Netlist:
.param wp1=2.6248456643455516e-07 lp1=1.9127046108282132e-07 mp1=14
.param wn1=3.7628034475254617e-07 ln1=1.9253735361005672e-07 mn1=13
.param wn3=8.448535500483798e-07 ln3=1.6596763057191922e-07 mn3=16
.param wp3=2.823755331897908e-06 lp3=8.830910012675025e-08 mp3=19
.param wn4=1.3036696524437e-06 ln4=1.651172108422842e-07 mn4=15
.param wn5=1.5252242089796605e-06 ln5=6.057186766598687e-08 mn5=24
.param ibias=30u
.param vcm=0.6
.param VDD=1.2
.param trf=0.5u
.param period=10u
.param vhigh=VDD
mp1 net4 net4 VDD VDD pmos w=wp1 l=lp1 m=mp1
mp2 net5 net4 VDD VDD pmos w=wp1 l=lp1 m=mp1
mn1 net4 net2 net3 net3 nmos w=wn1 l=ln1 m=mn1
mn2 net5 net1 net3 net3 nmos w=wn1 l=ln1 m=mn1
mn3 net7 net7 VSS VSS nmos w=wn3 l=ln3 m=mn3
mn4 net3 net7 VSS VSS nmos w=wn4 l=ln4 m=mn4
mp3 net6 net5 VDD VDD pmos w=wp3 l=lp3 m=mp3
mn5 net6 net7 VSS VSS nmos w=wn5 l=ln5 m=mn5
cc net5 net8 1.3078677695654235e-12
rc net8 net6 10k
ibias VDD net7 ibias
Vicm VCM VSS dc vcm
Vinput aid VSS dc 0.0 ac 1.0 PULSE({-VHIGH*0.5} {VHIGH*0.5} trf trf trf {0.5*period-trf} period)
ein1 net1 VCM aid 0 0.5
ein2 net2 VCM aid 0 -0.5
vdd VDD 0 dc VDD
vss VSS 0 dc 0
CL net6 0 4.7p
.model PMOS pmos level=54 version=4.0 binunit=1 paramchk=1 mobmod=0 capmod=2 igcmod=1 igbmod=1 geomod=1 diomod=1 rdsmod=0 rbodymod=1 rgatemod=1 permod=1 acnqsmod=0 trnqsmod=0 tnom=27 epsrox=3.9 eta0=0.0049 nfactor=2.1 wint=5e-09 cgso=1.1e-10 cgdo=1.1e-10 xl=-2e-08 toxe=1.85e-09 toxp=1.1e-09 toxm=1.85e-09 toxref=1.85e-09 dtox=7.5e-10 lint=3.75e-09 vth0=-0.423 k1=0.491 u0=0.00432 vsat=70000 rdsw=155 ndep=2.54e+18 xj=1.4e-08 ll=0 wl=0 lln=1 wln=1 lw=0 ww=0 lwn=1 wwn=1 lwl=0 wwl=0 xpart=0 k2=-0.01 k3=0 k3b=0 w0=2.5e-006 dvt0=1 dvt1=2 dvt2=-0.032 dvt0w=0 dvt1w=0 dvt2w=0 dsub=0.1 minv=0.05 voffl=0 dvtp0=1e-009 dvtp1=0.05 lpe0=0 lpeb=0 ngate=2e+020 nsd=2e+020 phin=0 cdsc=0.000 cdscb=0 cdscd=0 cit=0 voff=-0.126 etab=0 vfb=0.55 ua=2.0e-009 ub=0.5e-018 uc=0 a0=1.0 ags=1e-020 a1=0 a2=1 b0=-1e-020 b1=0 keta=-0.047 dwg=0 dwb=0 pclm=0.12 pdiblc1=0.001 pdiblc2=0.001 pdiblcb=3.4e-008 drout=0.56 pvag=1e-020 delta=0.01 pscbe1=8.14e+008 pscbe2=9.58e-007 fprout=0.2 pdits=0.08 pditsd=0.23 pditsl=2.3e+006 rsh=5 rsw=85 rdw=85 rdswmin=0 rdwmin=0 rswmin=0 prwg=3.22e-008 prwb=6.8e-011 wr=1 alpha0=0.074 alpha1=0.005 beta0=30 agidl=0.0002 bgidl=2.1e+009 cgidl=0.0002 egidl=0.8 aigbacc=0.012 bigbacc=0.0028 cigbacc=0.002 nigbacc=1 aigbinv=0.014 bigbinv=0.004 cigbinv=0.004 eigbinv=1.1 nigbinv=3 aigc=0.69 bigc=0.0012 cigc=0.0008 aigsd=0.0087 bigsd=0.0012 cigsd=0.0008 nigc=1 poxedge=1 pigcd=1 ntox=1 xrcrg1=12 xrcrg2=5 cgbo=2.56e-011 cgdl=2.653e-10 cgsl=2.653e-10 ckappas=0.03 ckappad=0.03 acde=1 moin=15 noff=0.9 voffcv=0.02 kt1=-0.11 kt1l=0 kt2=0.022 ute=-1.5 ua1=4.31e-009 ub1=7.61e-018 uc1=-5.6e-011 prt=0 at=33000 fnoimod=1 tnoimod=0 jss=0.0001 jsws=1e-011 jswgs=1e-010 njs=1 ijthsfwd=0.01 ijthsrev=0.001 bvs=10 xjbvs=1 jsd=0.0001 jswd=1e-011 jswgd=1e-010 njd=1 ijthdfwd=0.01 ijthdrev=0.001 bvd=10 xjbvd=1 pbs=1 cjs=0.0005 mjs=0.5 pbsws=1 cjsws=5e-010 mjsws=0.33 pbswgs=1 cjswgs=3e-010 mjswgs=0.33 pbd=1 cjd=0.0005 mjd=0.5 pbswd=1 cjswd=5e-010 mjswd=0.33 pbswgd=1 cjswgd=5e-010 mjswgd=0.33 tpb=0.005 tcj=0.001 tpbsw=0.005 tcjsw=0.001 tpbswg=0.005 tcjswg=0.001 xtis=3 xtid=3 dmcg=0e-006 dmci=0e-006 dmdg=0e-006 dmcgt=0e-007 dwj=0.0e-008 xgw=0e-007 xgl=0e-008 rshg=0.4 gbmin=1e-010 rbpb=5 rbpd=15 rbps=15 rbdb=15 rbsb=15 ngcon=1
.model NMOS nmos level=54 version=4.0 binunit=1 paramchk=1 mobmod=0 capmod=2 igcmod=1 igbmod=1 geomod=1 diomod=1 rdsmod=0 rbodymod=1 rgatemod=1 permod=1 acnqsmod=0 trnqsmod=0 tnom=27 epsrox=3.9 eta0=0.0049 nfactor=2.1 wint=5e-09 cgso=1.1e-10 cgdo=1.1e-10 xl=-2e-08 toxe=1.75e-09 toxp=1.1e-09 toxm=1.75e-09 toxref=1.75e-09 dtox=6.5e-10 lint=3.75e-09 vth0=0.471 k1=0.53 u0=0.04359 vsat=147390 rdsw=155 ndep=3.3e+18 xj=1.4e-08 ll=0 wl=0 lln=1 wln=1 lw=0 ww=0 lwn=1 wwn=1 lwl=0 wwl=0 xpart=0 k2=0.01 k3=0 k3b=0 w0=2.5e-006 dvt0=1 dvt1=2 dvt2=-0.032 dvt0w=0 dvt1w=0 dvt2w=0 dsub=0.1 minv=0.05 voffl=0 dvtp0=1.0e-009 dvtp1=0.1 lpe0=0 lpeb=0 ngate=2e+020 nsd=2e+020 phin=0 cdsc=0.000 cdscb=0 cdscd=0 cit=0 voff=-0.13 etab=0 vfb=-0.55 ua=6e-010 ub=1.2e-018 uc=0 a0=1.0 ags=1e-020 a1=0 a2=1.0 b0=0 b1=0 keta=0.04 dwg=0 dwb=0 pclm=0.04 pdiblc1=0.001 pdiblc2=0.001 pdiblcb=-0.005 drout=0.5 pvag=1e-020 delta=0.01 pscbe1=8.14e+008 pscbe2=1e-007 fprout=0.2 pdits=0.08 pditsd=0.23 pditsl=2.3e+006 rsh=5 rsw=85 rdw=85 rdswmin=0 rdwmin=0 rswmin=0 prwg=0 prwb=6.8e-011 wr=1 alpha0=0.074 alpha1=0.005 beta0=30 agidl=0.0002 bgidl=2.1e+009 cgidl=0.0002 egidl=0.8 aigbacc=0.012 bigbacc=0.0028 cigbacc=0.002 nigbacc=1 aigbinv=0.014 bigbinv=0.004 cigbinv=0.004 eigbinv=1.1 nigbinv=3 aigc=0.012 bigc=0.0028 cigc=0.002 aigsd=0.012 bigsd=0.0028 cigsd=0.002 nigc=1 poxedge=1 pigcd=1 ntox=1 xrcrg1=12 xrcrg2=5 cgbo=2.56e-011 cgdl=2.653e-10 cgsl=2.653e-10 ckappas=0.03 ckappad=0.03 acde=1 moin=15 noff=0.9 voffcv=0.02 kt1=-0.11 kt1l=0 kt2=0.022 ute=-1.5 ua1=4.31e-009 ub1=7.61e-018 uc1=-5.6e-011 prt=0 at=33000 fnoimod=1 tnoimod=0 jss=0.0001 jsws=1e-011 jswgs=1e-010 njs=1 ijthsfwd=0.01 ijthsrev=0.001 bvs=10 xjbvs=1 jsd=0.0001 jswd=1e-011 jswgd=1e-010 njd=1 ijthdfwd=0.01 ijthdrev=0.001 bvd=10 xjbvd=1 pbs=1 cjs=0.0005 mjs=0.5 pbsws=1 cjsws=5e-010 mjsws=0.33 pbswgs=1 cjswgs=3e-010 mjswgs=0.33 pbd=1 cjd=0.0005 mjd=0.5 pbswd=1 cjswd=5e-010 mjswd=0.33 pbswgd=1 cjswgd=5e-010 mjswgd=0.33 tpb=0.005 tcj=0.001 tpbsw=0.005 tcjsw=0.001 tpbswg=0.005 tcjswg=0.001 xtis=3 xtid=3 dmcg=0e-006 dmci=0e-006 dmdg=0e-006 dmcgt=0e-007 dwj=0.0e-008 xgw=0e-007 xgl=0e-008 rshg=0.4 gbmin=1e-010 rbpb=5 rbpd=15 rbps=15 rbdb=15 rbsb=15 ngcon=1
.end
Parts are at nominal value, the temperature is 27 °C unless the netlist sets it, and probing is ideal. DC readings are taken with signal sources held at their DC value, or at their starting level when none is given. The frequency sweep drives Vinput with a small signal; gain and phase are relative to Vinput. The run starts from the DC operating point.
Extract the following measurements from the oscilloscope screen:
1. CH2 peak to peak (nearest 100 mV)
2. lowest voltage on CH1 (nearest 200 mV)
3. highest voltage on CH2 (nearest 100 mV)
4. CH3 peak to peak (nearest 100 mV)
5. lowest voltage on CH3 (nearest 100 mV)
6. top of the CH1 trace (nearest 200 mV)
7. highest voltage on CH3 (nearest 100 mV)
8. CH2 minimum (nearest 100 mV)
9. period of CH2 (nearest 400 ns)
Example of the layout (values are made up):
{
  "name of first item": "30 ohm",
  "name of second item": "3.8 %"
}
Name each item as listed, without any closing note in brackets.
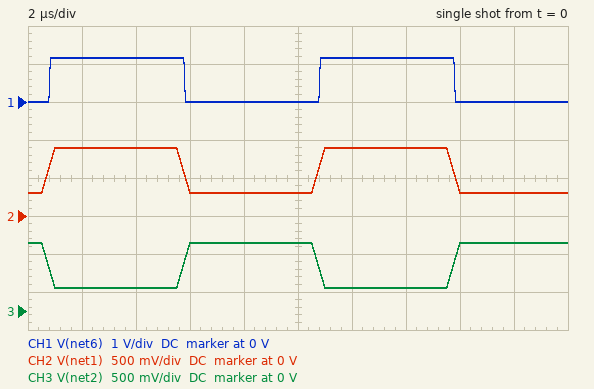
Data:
{
  "CH2 peak to peak": "600 mV",
  "lowest voltage on CH1": "0 V",
  "highest voltage on CH2": "900 mV",
  "CH3 peak to peak": "600 mV",
  "lowest voltage on CH3": "300 mV",
  "top of the CH1 trace": "1.2 V",
  "highest voltage on CH3": "900 mV",
  "CH2 minimum": "300 mV",
  "period of CH2": "10.0 µs"
}
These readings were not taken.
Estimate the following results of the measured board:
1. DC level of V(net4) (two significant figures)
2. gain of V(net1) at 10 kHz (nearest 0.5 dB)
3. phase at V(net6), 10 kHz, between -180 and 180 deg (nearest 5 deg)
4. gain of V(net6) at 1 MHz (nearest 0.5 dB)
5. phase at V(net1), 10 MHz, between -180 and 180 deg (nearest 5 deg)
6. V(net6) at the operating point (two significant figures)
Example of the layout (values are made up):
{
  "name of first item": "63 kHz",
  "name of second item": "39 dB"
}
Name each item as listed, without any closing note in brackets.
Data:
{
  "DC level of V(net4)": "570 mV",
  "gain of V(net1) at 10 kHz": "-6.0 dB",
  "phase at V(net6), 10 kHz, between -180 and 180 deg": "-5 deg",
  "gain of V(net6) at 1 MHz": "30.0 dB",
  "phase at V(net1), 10 MHz, between -180 and 180 deg": "0 deg",
  "V(net6) at the operating point": "1.0 V"
}
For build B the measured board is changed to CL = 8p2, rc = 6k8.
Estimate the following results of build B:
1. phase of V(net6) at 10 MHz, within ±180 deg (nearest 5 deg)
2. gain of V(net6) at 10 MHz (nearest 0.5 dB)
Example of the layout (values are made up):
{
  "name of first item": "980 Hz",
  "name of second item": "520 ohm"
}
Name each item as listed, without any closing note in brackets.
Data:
{
  "phase of V(net6) at 10 MHz, within ±180 deg": "-65 deg",
  "gain of V(net6) at 10 MHz": "11.0 dB"
}
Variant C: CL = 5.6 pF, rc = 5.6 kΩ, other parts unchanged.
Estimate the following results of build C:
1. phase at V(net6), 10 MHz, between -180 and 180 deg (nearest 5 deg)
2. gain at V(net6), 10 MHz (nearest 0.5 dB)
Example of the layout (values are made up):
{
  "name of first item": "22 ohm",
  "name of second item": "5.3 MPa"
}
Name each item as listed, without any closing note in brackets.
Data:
{
  "phase at V(net6), 10 MHz, between -180 and 180 deg": "-70 deg",
  "gain at V(net6), 10 MHz": "10.5 dB"
}
